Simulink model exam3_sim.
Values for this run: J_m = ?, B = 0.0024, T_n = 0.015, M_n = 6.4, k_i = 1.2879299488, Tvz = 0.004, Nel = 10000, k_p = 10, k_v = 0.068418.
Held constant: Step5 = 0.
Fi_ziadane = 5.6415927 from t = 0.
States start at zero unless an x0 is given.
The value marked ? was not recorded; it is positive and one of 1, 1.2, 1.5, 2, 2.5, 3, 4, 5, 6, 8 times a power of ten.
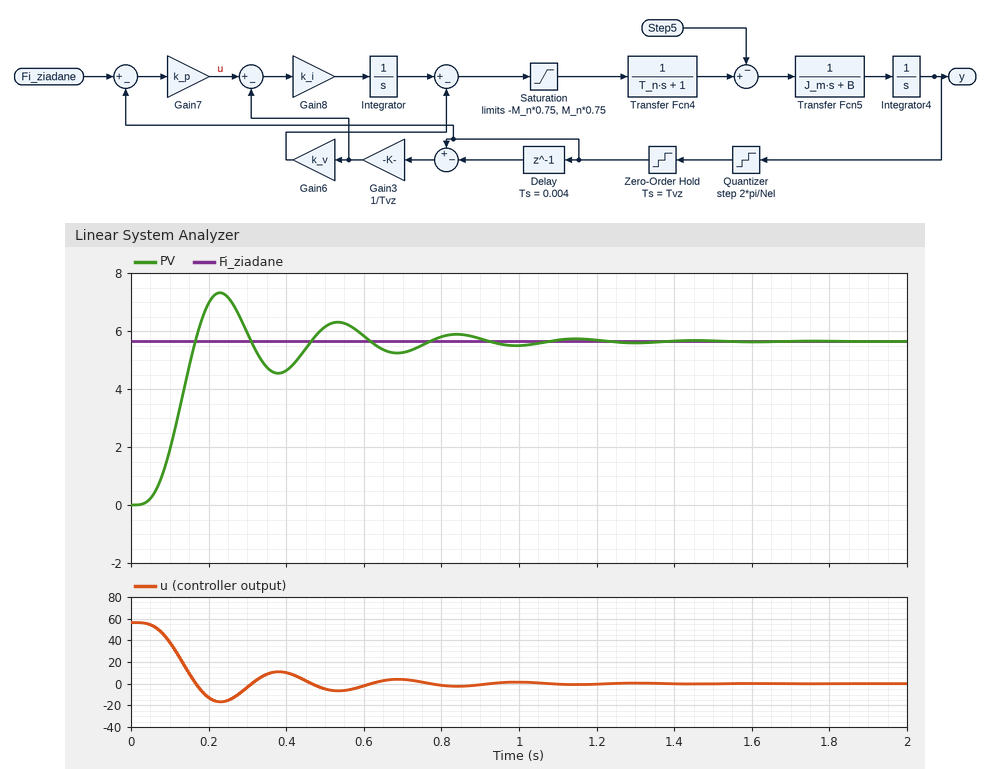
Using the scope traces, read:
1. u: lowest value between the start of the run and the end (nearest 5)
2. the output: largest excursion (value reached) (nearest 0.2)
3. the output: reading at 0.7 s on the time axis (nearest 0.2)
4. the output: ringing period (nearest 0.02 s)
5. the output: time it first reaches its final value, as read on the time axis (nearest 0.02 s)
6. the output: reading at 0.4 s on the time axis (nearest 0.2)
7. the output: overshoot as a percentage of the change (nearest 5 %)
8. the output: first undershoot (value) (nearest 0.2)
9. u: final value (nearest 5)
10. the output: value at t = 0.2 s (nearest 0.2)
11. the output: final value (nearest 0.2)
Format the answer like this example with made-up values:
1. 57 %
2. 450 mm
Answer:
1. -15
2. 7.4
3. 5.2
4. 0.30 s
5. 0.16 s
6. 4.6
7. 30 %
8. 4.6
9. 0
10. 7.0
11. 5.6
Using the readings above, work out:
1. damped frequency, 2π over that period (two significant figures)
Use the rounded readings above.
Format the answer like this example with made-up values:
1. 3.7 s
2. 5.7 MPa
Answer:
1. 21 rad/s
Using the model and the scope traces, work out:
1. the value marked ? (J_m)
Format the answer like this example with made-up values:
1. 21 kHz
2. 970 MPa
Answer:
1. 0.003
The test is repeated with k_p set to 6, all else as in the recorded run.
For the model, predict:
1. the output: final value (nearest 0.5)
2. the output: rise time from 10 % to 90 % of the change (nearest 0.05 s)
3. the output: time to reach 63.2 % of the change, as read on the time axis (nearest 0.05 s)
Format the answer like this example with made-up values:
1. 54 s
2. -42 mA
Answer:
1. 5.5
2. 0.15 s
3. 0.15 s
